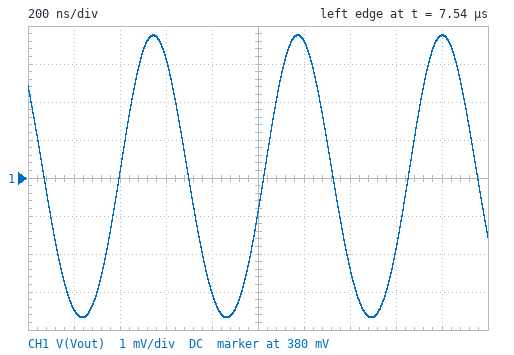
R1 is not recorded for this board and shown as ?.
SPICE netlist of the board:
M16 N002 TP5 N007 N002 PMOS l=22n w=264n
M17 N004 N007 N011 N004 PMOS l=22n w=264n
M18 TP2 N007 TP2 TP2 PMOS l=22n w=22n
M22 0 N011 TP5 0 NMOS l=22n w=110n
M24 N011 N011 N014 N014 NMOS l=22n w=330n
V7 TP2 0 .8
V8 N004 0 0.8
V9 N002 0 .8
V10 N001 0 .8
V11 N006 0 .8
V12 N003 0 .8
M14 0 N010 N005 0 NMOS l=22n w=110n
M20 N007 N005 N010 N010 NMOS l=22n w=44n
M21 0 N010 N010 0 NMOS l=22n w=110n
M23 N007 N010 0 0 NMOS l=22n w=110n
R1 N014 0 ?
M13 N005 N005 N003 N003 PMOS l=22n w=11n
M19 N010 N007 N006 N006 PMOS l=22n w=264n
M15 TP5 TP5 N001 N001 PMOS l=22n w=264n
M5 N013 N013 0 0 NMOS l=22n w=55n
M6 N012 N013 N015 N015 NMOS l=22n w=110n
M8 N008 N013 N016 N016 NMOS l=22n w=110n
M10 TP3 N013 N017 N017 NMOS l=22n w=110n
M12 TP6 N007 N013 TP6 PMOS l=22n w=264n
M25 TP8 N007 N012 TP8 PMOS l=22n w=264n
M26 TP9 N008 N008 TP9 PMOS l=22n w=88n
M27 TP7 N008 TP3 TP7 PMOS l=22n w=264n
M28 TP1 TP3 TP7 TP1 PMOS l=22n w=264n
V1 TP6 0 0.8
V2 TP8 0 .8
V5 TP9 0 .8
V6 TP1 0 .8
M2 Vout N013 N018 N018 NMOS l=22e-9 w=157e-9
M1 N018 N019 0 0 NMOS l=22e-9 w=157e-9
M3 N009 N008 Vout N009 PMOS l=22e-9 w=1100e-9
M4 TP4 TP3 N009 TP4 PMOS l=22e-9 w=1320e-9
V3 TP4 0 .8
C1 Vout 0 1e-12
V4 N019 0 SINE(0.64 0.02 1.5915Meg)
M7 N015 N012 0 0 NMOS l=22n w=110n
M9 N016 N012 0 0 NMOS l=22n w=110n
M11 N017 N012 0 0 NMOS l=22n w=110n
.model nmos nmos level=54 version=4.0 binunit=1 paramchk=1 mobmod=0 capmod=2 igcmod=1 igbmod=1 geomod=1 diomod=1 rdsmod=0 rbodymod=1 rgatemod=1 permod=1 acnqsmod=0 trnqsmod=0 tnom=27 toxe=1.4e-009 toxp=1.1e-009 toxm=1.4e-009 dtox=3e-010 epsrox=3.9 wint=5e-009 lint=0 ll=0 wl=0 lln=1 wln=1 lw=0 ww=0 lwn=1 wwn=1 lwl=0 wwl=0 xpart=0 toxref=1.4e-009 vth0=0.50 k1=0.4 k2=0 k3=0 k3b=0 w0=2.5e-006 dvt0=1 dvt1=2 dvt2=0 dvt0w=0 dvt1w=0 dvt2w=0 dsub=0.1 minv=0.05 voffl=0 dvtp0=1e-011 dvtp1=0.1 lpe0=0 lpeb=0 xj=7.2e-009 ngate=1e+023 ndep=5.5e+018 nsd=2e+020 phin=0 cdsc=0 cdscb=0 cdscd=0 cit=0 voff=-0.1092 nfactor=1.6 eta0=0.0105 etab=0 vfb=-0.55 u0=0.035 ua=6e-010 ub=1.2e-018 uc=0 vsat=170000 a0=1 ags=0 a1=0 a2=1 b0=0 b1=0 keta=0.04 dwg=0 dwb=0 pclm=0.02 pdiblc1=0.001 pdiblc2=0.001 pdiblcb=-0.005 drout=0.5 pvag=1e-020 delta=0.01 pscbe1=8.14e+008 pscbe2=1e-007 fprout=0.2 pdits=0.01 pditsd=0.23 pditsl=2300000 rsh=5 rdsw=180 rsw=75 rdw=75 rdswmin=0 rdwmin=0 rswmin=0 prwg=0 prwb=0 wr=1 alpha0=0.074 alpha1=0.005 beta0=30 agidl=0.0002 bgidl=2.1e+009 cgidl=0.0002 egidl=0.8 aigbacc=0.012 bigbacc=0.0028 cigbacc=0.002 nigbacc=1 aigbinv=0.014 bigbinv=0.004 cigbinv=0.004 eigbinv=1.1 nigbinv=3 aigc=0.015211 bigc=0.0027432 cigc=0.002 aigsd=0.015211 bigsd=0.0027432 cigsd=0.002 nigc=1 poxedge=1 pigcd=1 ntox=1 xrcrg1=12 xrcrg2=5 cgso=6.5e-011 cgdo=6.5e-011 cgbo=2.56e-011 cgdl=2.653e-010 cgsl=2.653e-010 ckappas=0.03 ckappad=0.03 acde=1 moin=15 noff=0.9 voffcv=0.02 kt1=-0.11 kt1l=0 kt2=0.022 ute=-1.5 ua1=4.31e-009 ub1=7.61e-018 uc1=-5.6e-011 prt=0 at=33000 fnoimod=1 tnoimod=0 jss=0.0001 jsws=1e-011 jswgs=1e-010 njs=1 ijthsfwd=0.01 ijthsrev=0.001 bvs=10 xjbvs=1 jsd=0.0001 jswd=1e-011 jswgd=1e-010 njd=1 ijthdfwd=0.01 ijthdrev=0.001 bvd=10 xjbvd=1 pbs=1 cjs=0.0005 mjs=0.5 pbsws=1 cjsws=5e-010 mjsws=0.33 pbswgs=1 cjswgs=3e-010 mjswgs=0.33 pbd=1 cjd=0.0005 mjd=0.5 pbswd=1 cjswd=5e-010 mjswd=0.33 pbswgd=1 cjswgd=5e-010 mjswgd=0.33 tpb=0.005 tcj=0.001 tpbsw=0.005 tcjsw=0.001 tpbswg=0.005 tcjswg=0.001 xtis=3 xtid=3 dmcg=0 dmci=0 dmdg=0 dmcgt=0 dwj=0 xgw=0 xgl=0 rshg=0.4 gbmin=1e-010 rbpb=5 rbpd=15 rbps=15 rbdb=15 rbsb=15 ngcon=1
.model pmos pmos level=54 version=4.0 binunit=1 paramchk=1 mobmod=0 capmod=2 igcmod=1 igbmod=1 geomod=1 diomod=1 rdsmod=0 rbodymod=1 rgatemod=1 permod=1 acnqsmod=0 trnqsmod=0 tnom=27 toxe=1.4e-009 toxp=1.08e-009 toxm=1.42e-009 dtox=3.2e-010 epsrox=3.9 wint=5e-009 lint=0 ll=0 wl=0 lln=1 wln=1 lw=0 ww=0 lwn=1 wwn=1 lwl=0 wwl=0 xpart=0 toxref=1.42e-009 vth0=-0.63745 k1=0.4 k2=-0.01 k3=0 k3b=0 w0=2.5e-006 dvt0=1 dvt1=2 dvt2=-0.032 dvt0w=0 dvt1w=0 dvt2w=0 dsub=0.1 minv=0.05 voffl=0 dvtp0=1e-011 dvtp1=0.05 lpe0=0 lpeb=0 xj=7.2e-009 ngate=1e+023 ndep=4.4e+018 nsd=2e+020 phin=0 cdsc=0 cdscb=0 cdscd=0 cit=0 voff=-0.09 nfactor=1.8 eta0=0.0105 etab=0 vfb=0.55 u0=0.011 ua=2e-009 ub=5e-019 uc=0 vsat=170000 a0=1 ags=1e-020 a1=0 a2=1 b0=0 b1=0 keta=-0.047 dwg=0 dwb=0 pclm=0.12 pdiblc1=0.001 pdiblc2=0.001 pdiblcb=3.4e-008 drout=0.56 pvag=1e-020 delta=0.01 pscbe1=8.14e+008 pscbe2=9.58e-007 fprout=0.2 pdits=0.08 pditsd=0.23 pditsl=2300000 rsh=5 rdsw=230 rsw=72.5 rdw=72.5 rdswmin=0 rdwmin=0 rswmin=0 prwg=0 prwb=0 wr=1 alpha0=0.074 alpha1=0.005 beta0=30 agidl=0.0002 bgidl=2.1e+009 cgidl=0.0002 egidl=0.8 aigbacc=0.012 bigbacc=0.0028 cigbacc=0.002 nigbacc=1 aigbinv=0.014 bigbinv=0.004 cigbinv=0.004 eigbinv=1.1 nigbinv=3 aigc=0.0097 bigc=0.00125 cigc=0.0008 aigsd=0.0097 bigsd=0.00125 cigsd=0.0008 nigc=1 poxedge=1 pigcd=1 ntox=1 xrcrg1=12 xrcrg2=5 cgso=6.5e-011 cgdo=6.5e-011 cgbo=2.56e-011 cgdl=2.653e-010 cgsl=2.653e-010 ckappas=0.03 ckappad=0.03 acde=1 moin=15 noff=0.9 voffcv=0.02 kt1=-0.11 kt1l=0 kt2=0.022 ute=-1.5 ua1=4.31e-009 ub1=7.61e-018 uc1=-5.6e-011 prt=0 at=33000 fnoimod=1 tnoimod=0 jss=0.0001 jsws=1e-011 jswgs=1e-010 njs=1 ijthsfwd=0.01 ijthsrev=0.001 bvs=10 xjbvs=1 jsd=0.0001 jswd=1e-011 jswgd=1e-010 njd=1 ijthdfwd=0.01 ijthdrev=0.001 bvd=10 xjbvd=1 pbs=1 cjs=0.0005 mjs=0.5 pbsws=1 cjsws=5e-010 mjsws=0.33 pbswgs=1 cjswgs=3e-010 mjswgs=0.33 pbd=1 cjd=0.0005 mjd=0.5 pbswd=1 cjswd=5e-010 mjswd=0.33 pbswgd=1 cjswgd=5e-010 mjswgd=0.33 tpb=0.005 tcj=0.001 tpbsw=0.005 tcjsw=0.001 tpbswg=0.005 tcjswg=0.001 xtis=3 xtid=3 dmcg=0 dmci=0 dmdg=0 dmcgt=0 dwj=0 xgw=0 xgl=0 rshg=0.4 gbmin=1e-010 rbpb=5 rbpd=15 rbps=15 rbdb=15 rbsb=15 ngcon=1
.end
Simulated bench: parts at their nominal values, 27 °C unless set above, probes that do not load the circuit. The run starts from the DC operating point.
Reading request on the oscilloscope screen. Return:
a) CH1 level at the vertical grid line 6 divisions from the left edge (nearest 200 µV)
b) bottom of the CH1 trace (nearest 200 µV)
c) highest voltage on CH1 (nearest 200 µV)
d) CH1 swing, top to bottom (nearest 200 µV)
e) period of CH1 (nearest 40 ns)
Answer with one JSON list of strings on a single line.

["383.6 mV", "376.4 mV", "383.8 mV", "7.4 mV", "640 ns"]
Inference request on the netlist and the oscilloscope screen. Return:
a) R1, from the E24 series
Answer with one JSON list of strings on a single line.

["16 kΩ"]
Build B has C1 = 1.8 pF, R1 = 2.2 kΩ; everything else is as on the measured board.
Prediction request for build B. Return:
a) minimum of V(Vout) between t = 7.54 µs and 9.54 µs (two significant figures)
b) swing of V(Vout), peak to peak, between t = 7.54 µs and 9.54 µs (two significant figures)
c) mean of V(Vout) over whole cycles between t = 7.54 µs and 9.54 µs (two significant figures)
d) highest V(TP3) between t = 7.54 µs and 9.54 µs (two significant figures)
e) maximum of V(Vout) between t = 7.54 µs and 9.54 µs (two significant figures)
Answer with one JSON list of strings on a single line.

["440 mV", "24 mV", "450 mV", "100 mV", "460 mV"]
